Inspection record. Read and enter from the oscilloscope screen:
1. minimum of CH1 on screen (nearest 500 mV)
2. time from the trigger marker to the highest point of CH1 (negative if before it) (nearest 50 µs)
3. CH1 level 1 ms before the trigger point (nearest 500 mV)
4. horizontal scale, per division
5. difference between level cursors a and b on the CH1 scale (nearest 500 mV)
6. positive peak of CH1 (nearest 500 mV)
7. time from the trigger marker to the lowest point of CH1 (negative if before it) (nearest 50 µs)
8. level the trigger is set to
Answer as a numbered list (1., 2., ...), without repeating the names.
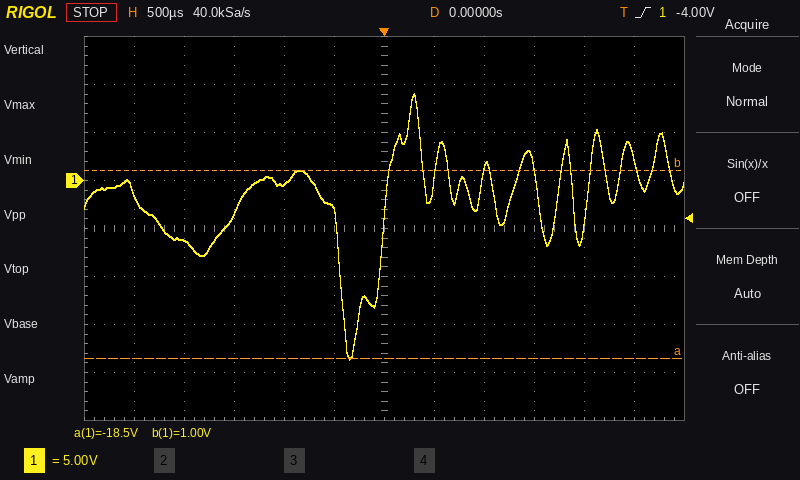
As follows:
1. -18.5 V
2. +300 µs
3. -500 mV
4. 500 µs
5. 19.5 V
6. 9.0 V
7. -350 µs
8. -4.00 V
